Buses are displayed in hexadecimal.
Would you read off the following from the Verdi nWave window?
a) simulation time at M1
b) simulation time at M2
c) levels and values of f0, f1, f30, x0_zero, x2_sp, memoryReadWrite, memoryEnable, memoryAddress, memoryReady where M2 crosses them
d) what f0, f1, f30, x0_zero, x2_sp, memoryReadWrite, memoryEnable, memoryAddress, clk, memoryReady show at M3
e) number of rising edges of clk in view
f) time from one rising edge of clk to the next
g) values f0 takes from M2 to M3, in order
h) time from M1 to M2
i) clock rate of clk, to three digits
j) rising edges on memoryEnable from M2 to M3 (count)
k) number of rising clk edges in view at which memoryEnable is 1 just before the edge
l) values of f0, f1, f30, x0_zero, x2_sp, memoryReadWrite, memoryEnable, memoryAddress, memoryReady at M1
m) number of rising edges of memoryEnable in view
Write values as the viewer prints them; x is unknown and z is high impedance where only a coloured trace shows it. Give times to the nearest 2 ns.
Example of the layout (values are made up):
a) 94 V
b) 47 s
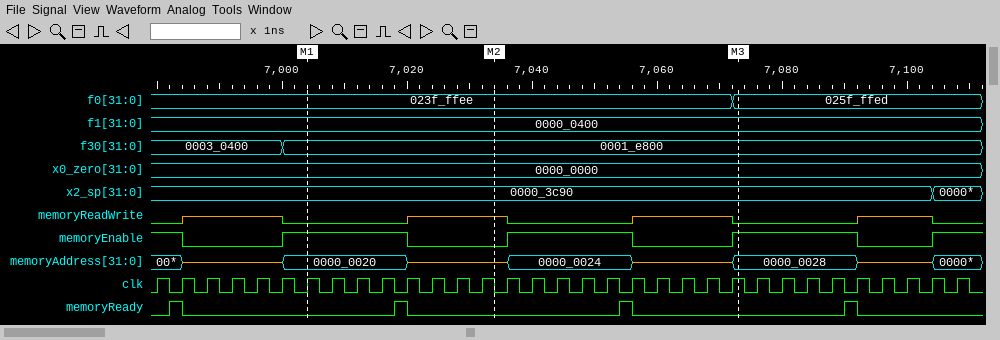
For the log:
a) 7004 ns
b) 7034 ns
c) f0=023f_ffee, f1=0000_0400, f30=0001_e800, x0_zero=0000_0000, x2_sp=0000_3c90, memoryReadWrite=z, memoryEnable=0, memoryAddress=z, memoryReady=0
d) f0=025f_ffed, f1=0000_0400, f30=0001_e800, x0_zero=0000_0000, x2_sp=0000_3c90, memoryReadWrite=0, memoryEnable=1, memoryAddress=0000_0028, clk=1, memoryReady=0
e) 33
f) 4 ns
g) 023f_ffee, 025f_ffed
h) 30 ns
i) 250 MHz
j) 2
k) 18
l) f0=023f_ffee, f1=0000_0400, f30=0001_e800, x0_zero=0000_0000, x2_sp=0000_3c90, memoryReadWrite=0, memoryEnable=1, memoryAddress=0000_0020, memoryReady=0
m) 4
